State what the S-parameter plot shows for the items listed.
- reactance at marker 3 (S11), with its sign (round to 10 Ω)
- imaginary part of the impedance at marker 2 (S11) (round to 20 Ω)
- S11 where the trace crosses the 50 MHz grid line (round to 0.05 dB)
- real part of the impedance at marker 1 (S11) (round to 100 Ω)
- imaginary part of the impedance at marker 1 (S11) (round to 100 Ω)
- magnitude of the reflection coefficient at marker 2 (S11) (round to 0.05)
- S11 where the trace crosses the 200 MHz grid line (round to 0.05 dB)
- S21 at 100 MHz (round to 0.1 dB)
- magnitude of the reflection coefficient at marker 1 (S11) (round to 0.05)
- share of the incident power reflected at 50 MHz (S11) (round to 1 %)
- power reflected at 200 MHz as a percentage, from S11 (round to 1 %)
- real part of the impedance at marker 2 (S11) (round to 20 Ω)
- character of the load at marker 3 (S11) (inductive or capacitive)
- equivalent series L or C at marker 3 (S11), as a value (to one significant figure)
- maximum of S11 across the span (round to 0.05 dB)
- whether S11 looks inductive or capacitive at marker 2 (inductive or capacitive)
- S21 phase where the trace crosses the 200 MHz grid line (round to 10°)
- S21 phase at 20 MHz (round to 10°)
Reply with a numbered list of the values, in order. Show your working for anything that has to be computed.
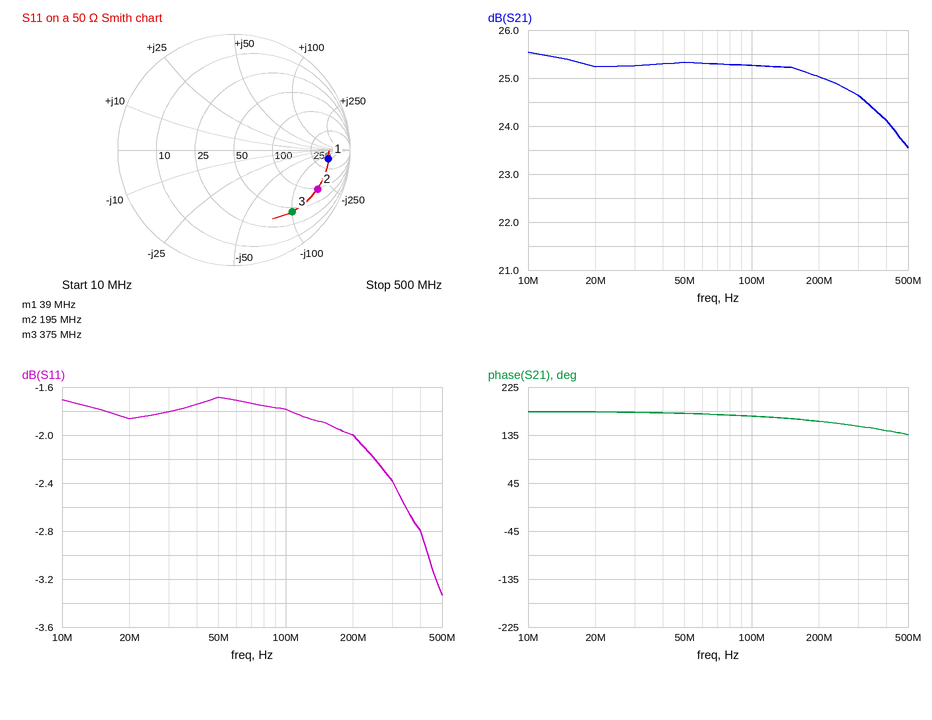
1. -100 Ω
2. -180 Ω
3. -1.70 dB
4. 400 Ω
5. -200 Ω
6. 0.80
7. -2.00 dB
8. 25.3 dB
9. 0.80
10. 10^(-1.7/10) ≈ 68 %
11. 10^(-2/10) ≈ 63 %
12. 100 Ω
13. capacitive
14. C = 1/(2π × 375 MHz × 100 Ω) ≈ 4 pF
15. -1.70 dB
16. capacitive
17. 160°
18. 180°
